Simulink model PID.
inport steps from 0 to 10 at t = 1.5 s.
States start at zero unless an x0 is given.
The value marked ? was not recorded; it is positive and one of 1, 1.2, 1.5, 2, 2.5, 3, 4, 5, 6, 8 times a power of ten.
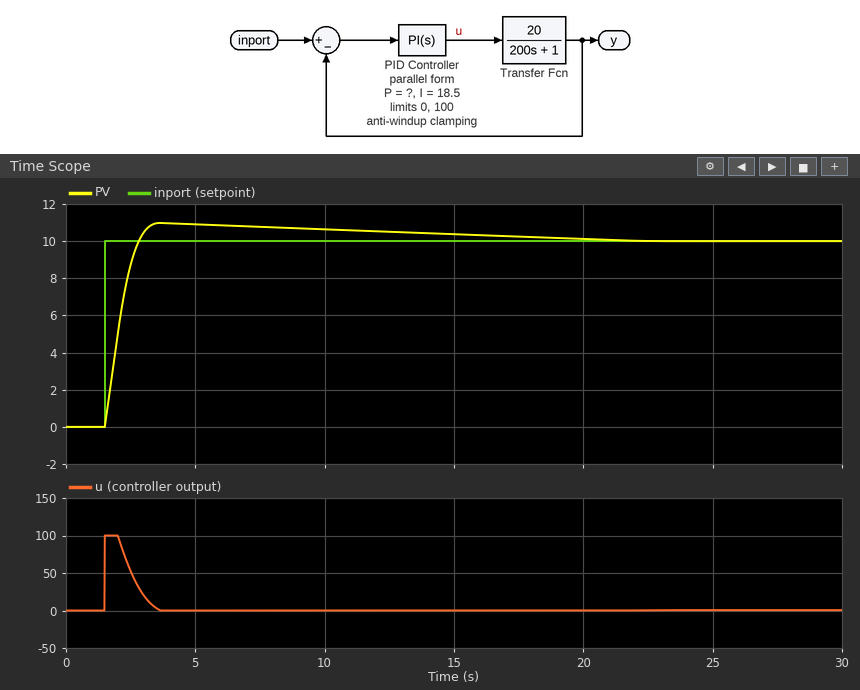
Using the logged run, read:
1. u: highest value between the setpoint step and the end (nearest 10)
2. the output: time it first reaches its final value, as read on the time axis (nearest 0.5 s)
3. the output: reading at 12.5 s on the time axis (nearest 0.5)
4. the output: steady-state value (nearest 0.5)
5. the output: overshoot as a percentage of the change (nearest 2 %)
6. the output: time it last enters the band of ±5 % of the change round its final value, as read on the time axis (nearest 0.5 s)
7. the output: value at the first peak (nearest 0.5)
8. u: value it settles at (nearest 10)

100
3.0 s
10.5
10.0
10 %
12.5 s
11.0
0
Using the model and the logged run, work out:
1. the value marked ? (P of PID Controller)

20
